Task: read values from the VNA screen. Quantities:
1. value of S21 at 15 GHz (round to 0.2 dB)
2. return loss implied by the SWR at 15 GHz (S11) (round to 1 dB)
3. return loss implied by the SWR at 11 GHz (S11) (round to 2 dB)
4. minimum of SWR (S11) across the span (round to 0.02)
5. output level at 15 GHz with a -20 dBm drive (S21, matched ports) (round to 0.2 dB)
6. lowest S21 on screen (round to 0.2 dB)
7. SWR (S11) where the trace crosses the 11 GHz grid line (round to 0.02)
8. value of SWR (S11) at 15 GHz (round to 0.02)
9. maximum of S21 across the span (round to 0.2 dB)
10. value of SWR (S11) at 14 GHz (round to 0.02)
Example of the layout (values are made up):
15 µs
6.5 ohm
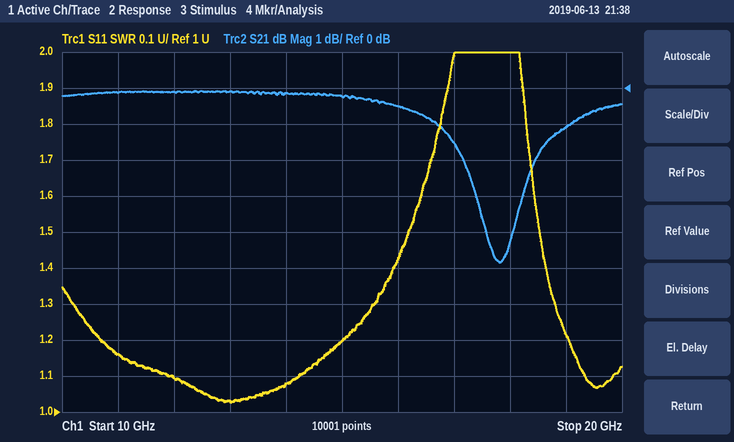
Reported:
-0.2 dB
21 dB
22 dB
1.02
-20.2 dBm
-4.8 dB
1.16
1.20
0.0 dB
1.08
